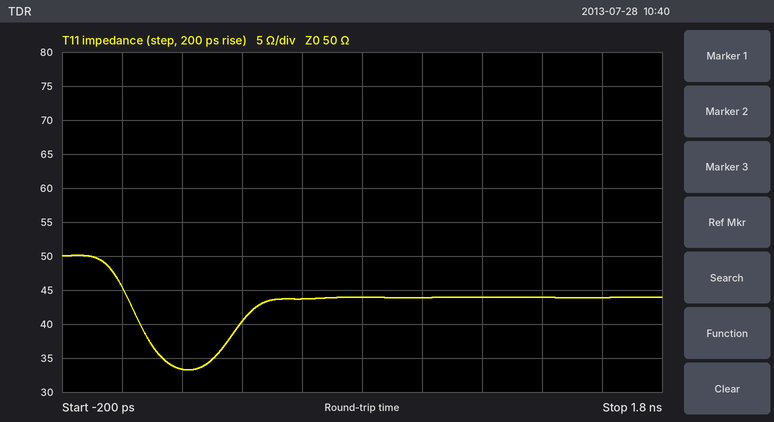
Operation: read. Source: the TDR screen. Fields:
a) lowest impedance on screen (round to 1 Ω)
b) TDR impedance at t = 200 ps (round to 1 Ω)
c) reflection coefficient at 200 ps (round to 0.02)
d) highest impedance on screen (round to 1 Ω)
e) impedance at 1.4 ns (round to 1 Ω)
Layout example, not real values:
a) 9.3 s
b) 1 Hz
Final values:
a) 33 Ω
b) 33 Ω
c) -0.20
d) 50 Ω
e) 44 Ω
